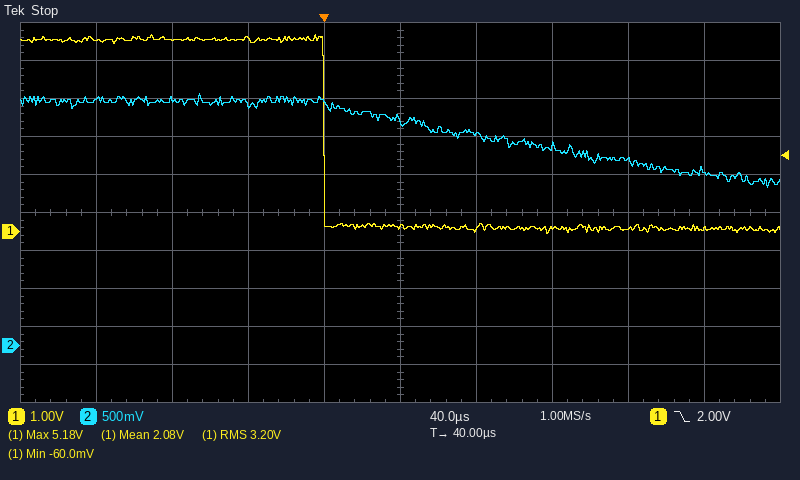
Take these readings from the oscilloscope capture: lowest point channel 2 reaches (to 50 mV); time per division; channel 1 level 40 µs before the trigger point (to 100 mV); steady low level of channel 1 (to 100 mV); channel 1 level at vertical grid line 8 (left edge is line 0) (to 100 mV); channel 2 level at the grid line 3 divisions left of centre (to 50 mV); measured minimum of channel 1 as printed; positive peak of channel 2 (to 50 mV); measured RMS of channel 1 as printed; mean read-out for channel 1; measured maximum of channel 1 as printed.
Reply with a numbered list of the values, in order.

1. 2.10 V
2. 40 µs
3. 5.1 V
4. 100 mV
5. 100 mV
6. 3.25 V
7. -60.0 mV
8. 3.30 V
9. 3.20 V
10. 2.08 V
11. 5.18 V
